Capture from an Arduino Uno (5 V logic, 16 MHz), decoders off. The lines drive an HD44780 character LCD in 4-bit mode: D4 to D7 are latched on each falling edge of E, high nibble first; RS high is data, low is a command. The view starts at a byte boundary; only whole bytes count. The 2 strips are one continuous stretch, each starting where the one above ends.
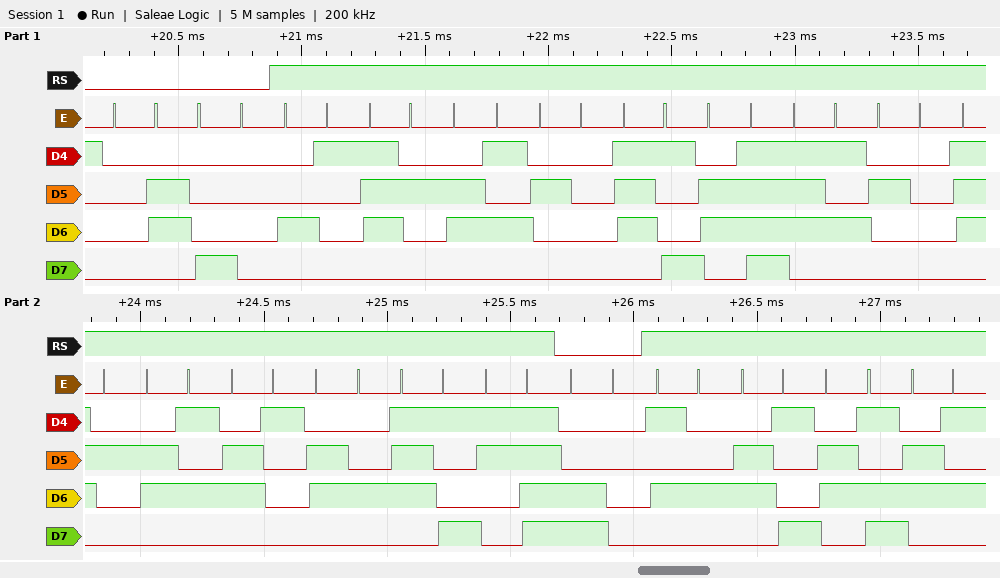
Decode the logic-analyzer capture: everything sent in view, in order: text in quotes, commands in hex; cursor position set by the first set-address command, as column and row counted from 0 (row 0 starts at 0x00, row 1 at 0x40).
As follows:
0x06 0x80 "Are you ready?" 0xC0 "Time"
column 0, row 0
